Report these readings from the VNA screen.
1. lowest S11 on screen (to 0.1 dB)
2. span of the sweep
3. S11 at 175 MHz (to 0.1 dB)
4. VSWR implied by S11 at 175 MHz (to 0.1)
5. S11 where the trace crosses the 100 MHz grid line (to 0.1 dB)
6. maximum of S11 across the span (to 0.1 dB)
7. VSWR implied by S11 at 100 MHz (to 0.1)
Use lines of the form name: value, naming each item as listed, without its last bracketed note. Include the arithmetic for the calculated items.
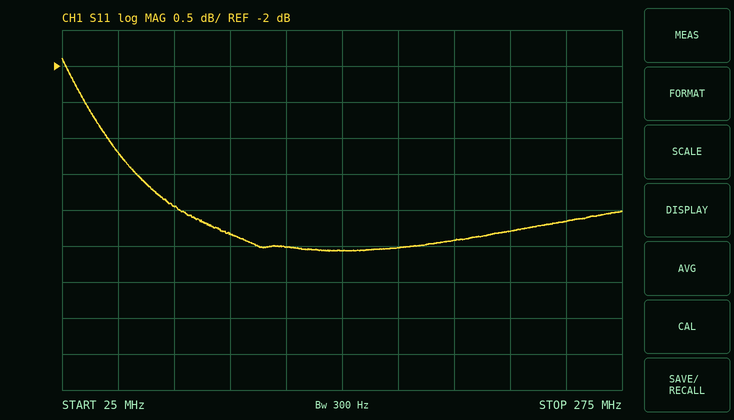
lowest S11 on screen: -4.6 dB
span of the sweep: 250 MHz
S11 at 175 MHz: -4.5 dB
VSWR implied by S11 at 175 MHz: |Γ| = 10^(-4.5/20) = 0.5957; VSWR = (1 + 0.5957)/(1 − 0.5957) ≈ 3.9
S11 where the trace crosses the 100 MHz grid line: -4.3 dB
maximum of S11 across the span: -1.9 dB
VSWR implied by S11 at 100 MHz: |Γ| = 10^(-4.3/20) = 0.6095; VSWR = (1 + 0.6095)/(1 − 0.6095) ≈ 4.1
